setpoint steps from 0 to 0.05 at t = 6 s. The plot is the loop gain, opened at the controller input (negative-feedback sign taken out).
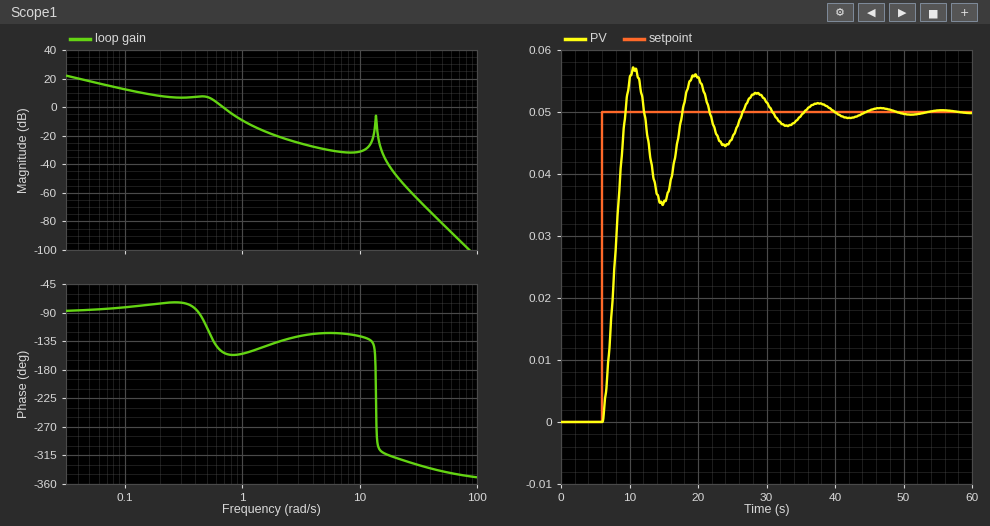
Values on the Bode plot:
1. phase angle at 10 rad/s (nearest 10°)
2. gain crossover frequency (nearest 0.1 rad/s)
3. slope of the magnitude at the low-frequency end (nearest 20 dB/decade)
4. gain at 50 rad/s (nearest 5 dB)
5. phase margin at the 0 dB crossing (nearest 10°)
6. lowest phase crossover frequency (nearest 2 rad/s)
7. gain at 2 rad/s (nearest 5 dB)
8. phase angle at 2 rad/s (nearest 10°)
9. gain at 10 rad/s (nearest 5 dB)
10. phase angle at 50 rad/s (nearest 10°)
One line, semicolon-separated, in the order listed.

-130°; 0.7 rad/s; -20 dB/decade; -80 dB; 30°; 14 rad/s; -20 dB; -140°; -30 dB; -340°
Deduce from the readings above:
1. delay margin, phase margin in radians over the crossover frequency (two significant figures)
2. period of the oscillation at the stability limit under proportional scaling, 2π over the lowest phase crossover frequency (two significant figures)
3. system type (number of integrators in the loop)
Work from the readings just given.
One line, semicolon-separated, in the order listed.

0.75 s; 0.45 s; 1
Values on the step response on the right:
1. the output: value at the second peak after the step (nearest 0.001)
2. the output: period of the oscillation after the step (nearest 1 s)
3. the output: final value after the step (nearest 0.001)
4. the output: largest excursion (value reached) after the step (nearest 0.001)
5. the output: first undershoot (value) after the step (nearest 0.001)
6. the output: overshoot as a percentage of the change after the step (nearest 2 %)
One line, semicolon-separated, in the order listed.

0.056; 9 s; 0.050; 0.057; 0.035; 14 %
